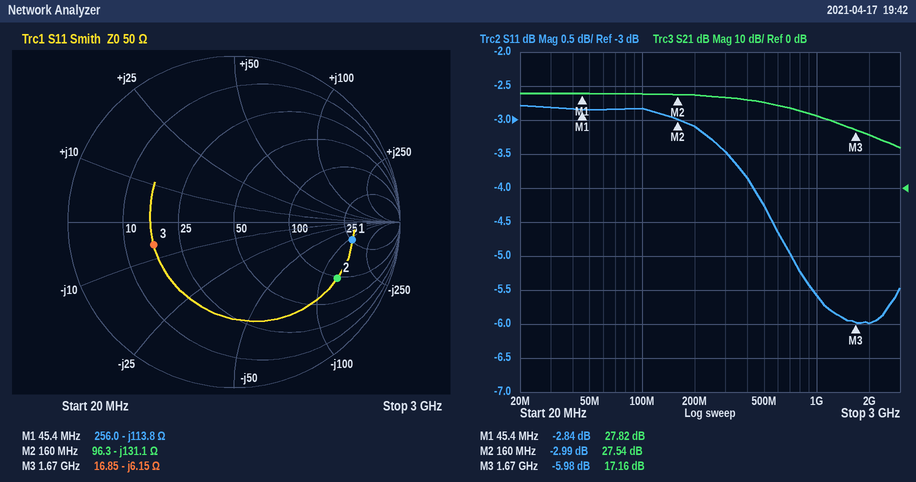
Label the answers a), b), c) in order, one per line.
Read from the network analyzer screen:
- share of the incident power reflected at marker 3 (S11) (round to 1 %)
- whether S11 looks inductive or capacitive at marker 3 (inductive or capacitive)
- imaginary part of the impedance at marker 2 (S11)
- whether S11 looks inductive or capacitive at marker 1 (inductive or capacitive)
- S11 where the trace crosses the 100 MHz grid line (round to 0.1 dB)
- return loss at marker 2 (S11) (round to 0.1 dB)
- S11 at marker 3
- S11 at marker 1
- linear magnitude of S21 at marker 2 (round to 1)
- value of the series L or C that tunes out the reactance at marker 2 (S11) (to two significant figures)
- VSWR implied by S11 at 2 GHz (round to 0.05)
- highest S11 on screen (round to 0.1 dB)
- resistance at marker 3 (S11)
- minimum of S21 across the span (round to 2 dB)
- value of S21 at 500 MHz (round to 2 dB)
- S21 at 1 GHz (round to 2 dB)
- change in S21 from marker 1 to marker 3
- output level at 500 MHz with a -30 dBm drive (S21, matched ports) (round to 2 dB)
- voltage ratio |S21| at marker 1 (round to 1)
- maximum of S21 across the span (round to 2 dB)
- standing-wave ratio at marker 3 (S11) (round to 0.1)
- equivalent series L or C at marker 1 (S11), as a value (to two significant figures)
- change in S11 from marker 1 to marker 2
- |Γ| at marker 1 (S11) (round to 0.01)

a) 25 %
b) capacitive
c) -131.1 Ω
d) capacitive
e) -2.8 dB
f) 3.0 dB
g) -5.98 dB
h) -2.84 dB
i) 24
j) 130 nH
k) 3.00
l) -2.8 dB
m) 16.85 Ω
n) 12 dB
o) 26 dB
p) 22 dB
q) -10.66 dB
r) -4 dBm
s) 25
t) 28 dB
u) 3.0
v) 31 pF
w) -0.15 dB
x) 0.72
